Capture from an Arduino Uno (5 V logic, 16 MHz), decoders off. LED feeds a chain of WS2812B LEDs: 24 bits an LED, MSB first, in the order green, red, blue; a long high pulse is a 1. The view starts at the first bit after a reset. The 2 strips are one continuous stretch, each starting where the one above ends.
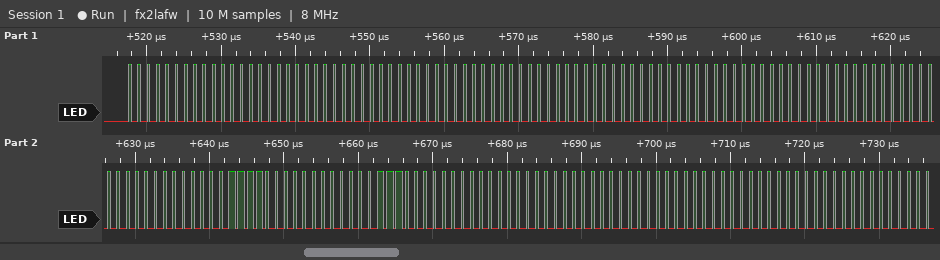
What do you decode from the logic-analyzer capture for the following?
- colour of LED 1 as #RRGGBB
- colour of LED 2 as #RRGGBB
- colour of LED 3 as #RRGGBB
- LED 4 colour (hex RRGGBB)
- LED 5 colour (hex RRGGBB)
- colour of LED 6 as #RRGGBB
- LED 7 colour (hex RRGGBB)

#000000
#000000
#000000
#000000
#000F0E
#000000
#000000
